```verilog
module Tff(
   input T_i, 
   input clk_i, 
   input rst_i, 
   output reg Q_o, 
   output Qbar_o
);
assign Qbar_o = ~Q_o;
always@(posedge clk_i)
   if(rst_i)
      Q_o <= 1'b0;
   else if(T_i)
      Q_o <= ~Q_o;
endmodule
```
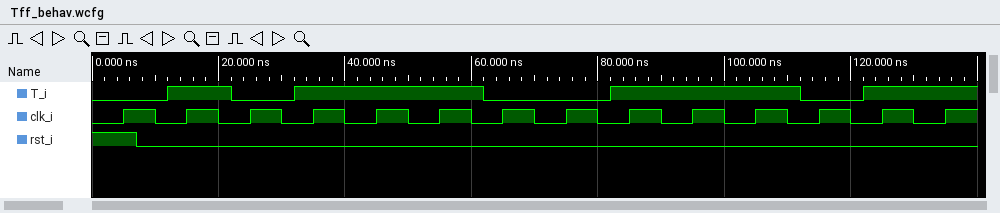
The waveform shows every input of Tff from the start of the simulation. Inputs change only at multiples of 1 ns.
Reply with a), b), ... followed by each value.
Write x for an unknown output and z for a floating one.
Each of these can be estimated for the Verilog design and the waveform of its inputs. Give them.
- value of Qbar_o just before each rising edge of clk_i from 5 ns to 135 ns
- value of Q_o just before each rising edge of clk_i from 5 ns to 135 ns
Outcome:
a) x 1 0 0 1 0 1 1 1 0 1 0 0 1
b) x 0 1 1 0 1 0 0 0 1 0 1 1 0
